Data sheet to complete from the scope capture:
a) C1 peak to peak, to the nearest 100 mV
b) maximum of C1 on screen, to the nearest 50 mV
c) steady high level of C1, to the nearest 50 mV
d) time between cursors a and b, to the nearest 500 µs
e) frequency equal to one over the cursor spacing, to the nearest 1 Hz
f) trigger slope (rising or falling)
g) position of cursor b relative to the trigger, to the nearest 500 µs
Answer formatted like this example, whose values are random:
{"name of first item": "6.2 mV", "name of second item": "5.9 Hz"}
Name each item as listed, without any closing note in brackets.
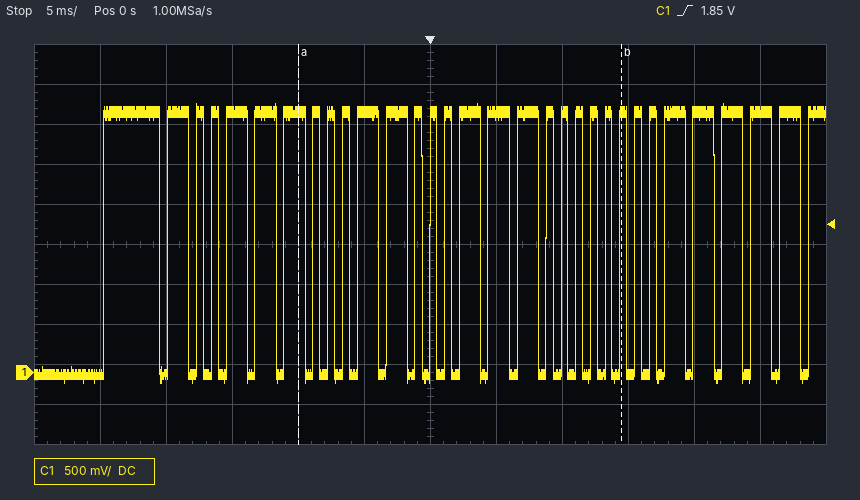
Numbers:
{"C1 peak to peak, to the nearest 100 mV": "3.50 V", "maximum of C1 on screen, to the nearest 50 mV": "3.35 V", "steady high level of C1, to the nearest 50 mV": "3.25 V", "time between cursors a and b, to the nearest 500 µs": "24.5 ms", "frequency equal to one over the cursor spacing, to the nearest 1 Hz": "41 Hz", "trigger slope": "rising", "position of cursor b relative to the trigger, to the nearest 500 µs": "+14.5 ms"}
